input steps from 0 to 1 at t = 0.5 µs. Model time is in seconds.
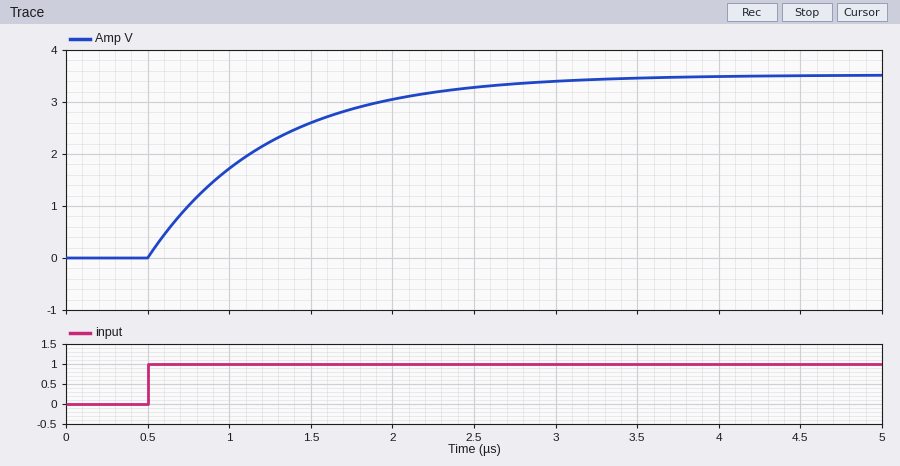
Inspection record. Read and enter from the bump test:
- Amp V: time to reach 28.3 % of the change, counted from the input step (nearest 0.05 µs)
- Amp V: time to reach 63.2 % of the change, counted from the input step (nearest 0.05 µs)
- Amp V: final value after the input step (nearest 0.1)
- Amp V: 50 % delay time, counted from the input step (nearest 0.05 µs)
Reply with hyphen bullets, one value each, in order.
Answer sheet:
- 0.25 µs
- 0.75 µs
- 3.5
- 0.50 µs
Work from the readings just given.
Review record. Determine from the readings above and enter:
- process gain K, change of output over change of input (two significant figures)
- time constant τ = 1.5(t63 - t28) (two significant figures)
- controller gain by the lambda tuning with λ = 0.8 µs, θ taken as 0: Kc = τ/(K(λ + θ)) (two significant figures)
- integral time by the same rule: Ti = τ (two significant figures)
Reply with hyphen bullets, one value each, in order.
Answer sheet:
- 3.5
- 0.75 µs
- 0.27
- 0.75 µs
